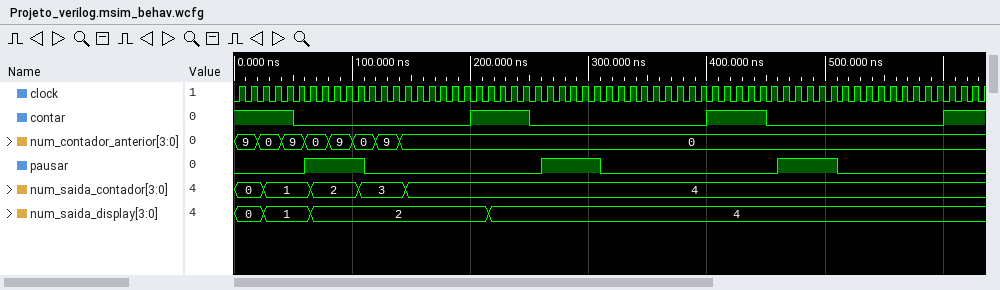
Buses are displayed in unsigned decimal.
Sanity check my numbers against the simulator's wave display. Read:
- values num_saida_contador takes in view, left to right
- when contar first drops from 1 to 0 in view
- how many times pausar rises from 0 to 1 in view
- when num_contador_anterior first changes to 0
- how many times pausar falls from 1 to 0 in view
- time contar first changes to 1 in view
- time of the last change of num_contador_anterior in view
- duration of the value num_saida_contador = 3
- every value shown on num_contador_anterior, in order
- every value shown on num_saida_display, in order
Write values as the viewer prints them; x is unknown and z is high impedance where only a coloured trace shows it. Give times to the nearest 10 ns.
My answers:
0, 1, 2, 3, 4
50 ns
3
20 ns
3
200 ns
140 ns
40 ns
9, 0, 9, 0, 9, 0, 9, 0
0, 1, 2, 4
